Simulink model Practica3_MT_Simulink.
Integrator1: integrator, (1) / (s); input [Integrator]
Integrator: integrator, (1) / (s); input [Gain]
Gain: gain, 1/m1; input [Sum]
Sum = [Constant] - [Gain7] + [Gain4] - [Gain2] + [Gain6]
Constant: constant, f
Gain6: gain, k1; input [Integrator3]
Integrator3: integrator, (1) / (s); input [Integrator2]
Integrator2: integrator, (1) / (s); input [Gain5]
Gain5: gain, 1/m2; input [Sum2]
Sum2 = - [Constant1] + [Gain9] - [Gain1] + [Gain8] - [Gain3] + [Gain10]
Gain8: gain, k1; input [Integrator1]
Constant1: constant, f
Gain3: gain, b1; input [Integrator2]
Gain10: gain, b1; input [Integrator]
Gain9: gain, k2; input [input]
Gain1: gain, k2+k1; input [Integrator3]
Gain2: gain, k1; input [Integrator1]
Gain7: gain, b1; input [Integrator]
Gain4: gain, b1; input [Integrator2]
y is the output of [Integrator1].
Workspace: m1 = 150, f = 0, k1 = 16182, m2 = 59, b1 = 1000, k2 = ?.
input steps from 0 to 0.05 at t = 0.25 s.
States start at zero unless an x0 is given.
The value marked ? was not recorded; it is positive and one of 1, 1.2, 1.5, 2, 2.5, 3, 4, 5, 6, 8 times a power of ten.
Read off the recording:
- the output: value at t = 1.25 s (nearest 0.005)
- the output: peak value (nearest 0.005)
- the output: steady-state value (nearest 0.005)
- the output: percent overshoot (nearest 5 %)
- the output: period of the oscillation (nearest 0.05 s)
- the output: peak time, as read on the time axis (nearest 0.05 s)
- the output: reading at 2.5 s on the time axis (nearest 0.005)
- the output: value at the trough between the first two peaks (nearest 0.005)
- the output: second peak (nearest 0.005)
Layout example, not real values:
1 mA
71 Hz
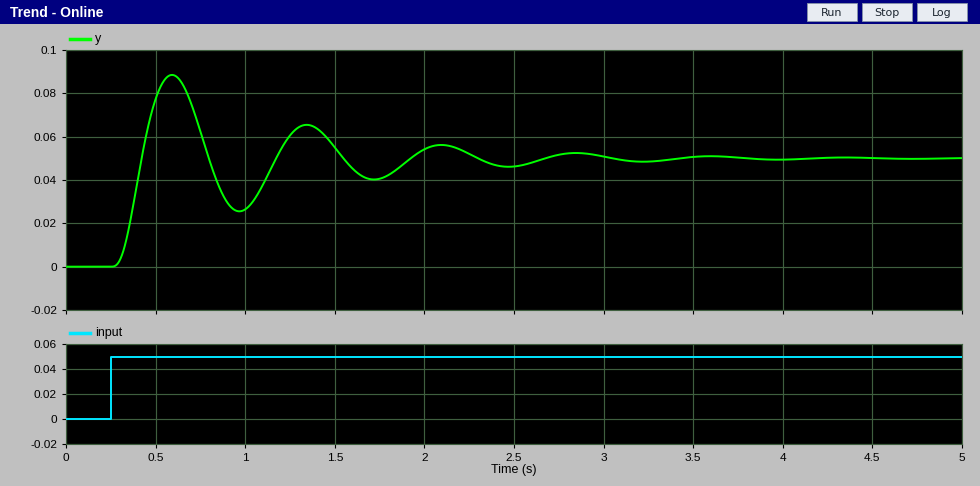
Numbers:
0.060
0.090
0.050
75 %
0.75 s
0.60 s
0.045
0.025
0.065
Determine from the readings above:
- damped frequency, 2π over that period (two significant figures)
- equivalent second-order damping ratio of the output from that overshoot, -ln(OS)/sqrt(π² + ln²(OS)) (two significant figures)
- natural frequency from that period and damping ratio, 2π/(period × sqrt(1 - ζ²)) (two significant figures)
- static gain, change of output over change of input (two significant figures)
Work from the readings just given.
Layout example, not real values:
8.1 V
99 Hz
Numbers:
8.4 rad/s
0.091
8.4 rad/s
1.0
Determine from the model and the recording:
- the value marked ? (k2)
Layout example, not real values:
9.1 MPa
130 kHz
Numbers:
30000
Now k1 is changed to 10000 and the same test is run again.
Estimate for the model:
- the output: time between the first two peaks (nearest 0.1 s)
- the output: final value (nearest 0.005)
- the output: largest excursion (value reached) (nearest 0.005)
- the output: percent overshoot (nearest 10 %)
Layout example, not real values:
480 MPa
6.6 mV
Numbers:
0.9 s
0.050
0.080
60 %
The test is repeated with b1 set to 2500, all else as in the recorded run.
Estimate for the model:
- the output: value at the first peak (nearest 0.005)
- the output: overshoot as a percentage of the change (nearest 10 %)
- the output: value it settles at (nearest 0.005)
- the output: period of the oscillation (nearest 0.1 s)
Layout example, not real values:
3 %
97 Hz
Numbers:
0.085
70 %
0.050
0.6 s
